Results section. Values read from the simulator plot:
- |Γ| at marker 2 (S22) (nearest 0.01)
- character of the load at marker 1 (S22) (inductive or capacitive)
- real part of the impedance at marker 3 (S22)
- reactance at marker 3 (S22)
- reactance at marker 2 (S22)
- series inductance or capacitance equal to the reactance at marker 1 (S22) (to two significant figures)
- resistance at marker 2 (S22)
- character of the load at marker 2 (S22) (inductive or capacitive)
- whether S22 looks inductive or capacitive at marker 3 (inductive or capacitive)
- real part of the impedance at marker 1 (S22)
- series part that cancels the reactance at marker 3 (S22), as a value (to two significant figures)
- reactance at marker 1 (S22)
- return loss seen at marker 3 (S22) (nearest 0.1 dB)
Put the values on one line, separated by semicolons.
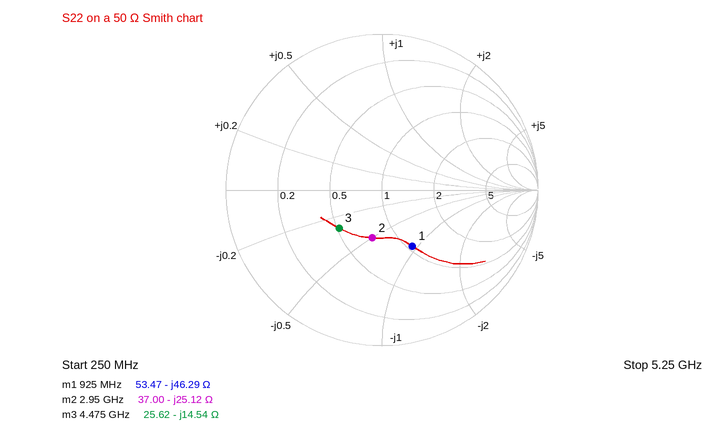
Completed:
0.31; capacitive; 25.62 Ω; -14.54 Ω; -25.12 Ω; 3.7 pF; 37.00 Ω; capacitive; capacitive; 53.47 Ω; 520 pH; -46.29 Ω; 8.7 dB
